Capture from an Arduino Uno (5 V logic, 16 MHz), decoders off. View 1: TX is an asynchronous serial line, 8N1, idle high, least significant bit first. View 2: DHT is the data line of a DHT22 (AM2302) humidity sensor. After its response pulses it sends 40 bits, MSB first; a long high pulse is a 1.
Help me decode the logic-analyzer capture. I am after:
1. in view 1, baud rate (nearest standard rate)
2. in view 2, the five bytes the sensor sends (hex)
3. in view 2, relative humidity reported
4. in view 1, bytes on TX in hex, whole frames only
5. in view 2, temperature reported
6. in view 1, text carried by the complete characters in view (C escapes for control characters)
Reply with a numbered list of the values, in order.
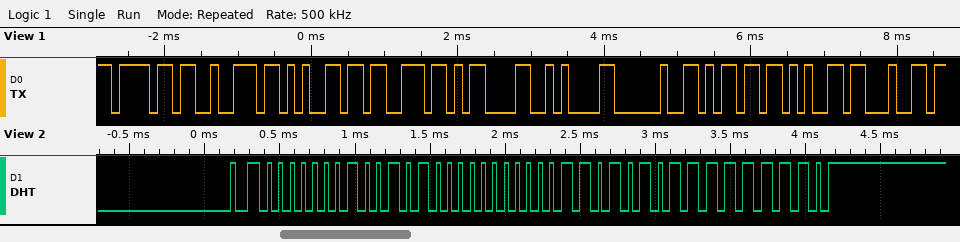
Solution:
1. 9600 baud
2. 01 28 00 D5 FE
3. 29.6 %
4. 6F 72 65 73 0D 0A 20 6D 65 64
5. 21.3 °C
6. "ores\r\n med"
